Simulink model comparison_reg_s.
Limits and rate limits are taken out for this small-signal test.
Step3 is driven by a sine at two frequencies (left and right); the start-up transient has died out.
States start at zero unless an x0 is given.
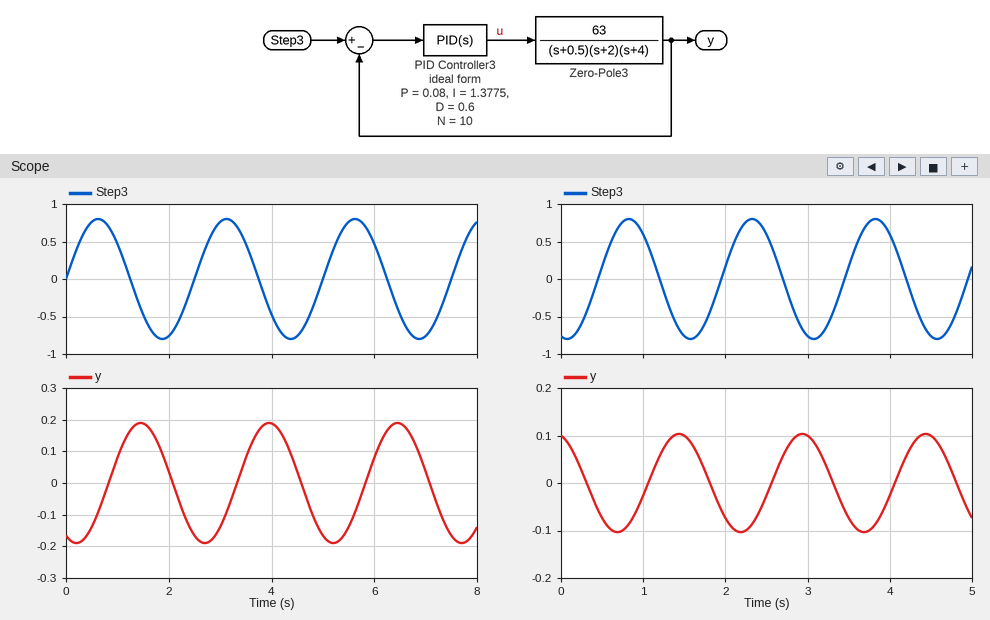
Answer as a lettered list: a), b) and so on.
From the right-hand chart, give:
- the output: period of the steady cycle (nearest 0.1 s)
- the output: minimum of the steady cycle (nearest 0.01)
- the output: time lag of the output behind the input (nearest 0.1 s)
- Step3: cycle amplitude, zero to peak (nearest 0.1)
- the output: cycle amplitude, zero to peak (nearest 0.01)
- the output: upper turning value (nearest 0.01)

a) 1.5 s
b) -0.10
c) 0.6 s
d) 0.8
e) 0.10
f) 0.10
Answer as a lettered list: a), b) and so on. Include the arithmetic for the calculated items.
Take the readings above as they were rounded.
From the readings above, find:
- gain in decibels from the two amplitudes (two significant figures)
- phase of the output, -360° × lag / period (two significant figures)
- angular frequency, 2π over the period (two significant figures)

a) 20 log10(0.1 / 0.8) = -18 dB
b) -360 × 0.6 / 1.5 = -140°
c) 2π / 1.5 = 4.2 rad/s
